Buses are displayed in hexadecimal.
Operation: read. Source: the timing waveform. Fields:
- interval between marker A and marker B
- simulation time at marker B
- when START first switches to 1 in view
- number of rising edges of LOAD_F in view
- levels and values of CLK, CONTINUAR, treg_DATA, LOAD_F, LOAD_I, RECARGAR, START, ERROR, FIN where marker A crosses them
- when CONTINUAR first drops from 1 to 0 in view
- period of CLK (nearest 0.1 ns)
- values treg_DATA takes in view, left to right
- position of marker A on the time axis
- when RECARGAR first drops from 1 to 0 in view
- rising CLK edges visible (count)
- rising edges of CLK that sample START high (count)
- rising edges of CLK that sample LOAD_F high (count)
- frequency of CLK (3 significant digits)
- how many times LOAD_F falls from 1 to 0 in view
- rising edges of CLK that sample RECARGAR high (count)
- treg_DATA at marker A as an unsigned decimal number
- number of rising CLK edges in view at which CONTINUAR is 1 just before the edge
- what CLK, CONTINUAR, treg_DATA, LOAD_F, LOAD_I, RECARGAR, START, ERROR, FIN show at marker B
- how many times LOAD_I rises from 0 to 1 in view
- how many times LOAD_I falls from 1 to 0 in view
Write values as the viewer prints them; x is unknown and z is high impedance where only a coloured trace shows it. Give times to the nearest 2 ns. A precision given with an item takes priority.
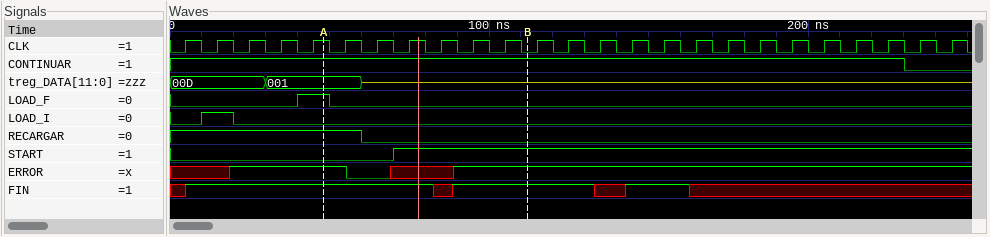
64 ns
112 ns
70 ns
1
CLK=1, CONTINUAR=1, treg_DATA=001, LOAD_F=1, LOAD_I=0, RECARGAR=1, START=0, ERROR=1, FIN=1
230 ns
10 ns
00D, 001, z
48 ns
60 ns
25
18
1
100 MHz
1
6
1
23
CLK=0, CONTINUAR=1, treg_DATA=z, LOAD_F=0, LOAD_I=0, RECARGAR=0, START=1, ERROR=1, FIN=1
1
1
